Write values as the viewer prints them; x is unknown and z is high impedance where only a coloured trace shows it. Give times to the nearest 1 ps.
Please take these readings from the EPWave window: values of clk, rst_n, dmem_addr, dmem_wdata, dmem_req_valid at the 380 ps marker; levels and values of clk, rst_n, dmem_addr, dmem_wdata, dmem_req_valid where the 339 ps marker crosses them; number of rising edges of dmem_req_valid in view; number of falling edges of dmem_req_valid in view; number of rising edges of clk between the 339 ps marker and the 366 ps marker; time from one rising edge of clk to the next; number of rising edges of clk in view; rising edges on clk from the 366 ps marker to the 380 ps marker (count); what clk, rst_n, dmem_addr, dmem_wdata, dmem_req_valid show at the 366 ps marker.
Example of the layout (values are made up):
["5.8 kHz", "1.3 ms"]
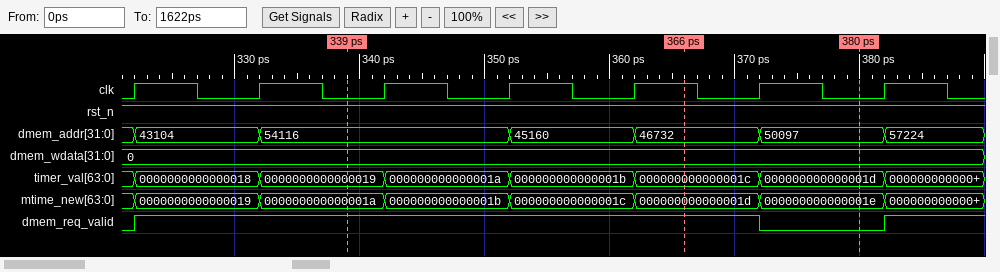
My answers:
["clk=0, rst_n=1, dmem_addr=50097, dmem_wdata=0, dmem_req_valid=0", "clk=0, rst_n=1, dmem_addr=54116, dmem_wdata=0, dmem_req_valid=1", "2", "1", "3", "10 ps", "7", "1", "clk=1, rst_n=1, dmem_addr=46732, dmem_wdata=0, dmem_req_valid=1"]
